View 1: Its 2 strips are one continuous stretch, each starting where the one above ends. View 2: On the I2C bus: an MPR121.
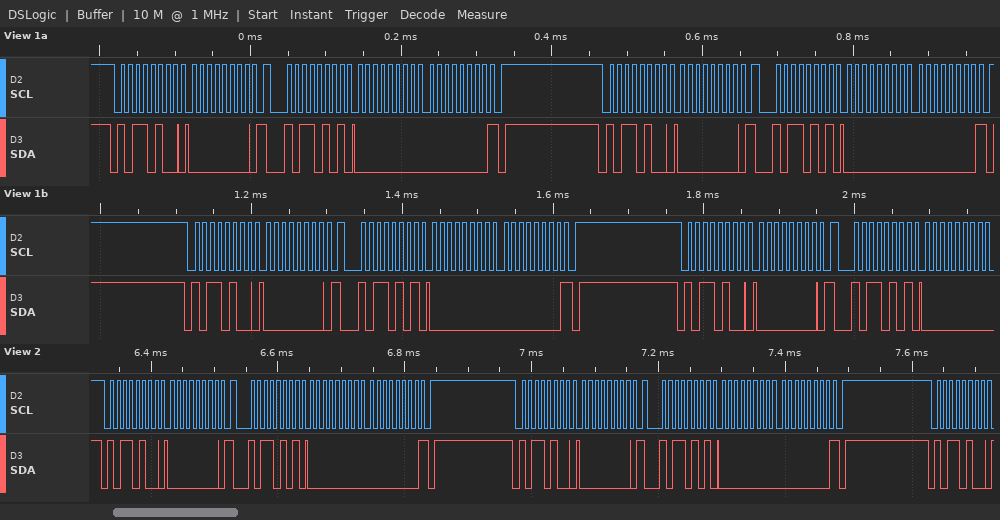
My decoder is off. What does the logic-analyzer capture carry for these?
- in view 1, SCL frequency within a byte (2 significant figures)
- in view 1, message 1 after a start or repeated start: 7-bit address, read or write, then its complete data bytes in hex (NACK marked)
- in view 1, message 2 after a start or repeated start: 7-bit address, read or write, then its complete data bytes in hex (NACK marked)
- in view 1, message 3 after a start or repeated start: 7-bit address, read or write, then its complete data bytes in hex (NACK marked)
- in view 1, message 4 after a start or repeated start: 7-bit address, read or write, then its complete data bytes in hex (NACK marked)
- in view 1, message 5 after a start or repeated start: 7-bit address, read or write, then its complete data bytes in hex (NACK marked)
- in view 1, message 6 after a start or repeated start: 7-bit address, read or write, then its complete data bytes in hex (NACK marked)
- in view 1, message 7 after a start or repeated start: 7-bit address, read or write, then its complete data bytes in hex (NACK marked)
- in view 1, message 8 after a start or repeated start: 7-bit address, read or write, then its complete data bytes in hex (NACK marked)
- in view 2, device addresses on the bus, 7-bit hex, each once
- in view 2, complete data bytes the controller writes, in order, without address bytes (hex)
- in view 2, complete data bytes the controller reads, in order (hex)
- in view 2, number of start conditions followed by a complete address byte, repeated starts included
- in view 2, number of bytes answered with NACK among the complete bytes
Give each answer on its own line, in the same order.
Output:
100 kHz
0x5A write: 00
0x5A read: 00 00 NACK
0x5A write: 00
0x5A read: 00 00 NACK
0x5A write: 00
0x5A read: 00 00 NACK
0x5A write: 00
0x5A read: 00
0x5A
00 00
00 00 00 00
5
2
